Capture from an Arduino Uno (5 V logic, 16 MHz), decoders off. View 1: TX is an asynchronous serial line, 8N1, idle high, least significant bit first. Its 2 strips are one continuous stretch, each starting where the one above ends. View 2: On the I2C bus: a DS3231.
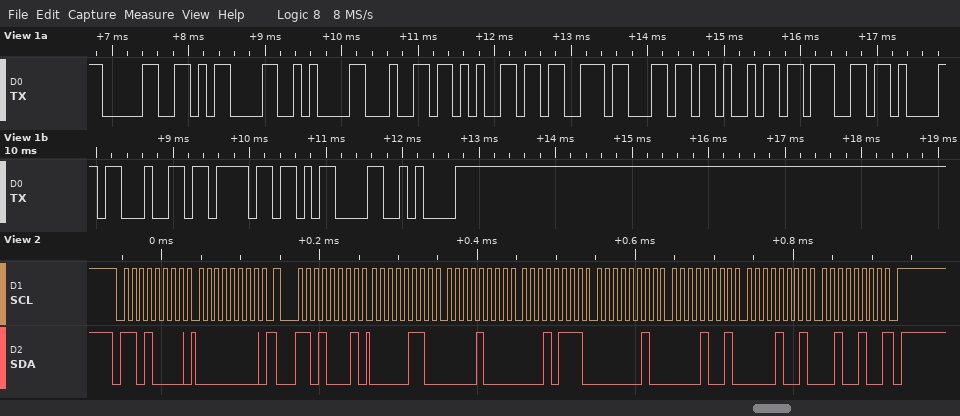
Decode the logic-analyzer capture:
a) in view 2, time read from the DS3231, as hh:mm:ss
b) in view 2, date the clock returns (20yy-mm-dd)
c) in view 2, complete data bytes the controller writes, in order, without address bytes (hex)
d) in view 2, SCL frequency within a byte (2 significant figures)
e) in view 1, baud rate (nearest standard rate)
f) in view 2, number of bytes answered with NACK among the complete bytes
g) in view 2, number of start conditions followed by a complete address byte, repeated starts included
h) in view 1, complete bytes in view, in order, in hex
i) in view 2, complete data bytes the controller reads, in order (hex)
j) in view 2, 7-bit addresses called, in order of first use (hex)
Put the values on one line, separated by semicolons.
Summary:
17:08:06; 2024-09-09; 00; 100 kHz; 9600 baud; 1; 2; 30 0D 0A 64 65 73 6C 69 67 61 64 6F 0D 0A; 06 08 17 02 09 09 24; 0x68
